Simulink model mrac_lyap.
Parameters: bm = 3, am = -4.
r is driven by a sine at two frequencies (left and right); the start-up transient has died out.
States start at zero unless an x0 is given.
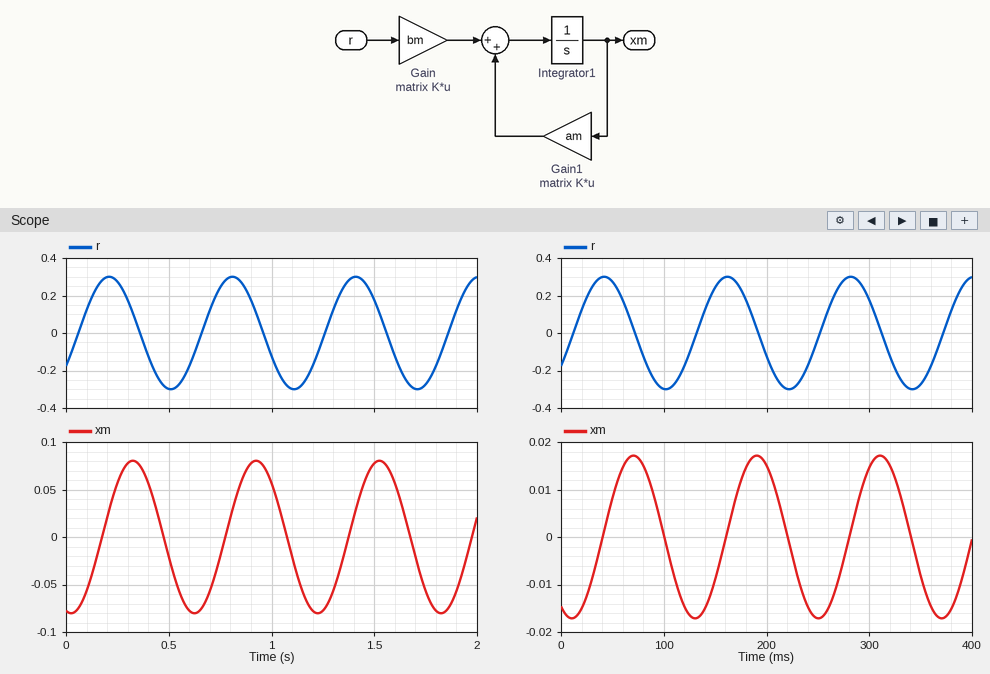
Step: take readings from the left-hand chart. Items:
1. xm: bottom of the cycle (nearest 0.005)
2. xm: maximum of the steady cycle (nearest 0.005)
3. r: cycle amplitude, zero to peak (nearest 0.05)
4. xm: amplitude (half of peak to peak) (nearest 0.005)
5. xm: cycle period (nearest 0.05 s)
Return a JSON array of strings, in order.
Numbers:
["-0.080", "0.080", "0.30", "0.080", "0.60 s"]
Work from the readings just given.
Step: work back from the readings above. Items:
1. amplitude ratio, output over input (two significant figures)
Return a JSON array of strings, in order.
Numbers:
["0.27"]
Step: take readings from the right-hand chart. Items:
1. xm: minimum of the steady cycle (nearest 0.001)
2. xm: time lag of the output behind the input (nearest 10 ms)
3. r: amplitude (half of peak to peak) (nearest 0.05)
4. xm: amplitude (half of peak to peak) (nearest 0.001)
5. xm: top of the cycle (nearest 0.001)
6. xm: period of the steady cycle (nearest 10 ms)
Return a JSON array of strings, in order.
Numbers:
["-0.017", "30 ms", "0.30", "0.017", "0.017", "120 ms"]
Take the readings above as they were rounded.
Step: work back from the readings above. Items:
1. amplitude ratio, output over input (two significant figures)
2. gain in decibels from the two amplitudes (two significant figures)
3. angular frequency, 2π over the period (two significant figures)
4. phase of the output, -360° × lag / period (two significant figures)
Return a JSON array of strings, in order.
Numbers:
["0.057", "-25 dB", "0.052 rad/ms", "-90°"]
